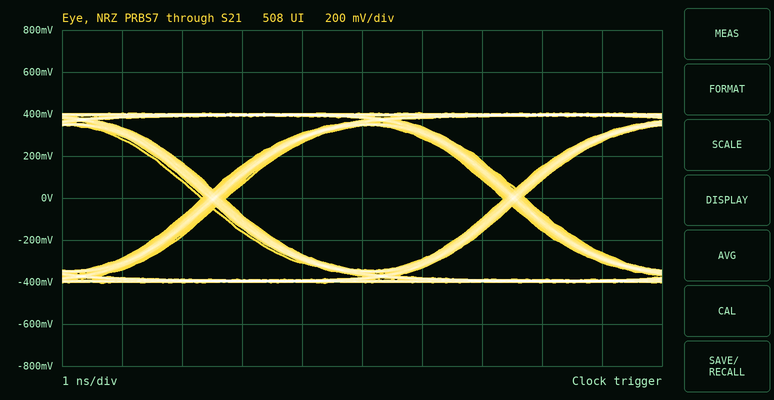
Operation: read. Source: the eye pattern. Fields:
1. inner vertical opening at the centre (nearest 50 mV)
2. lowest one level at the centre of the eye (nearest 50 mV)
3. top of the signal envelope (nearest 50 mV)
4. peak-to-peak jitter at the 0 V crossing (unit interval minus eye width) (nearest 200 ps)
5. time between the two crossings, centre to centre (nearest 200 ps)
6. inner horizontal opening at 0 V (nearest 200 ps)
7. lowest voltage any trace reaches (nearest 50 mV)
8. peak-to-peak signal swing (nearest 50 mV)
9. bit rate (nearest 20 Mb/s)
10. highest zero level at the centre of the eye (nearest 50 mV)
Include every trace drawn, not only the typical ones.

700 mV
350 mV
400 mV
400 ps
5.0 ns
4.6 ns
-400 mV
800 mV
200 Mb/s
-350 mV
